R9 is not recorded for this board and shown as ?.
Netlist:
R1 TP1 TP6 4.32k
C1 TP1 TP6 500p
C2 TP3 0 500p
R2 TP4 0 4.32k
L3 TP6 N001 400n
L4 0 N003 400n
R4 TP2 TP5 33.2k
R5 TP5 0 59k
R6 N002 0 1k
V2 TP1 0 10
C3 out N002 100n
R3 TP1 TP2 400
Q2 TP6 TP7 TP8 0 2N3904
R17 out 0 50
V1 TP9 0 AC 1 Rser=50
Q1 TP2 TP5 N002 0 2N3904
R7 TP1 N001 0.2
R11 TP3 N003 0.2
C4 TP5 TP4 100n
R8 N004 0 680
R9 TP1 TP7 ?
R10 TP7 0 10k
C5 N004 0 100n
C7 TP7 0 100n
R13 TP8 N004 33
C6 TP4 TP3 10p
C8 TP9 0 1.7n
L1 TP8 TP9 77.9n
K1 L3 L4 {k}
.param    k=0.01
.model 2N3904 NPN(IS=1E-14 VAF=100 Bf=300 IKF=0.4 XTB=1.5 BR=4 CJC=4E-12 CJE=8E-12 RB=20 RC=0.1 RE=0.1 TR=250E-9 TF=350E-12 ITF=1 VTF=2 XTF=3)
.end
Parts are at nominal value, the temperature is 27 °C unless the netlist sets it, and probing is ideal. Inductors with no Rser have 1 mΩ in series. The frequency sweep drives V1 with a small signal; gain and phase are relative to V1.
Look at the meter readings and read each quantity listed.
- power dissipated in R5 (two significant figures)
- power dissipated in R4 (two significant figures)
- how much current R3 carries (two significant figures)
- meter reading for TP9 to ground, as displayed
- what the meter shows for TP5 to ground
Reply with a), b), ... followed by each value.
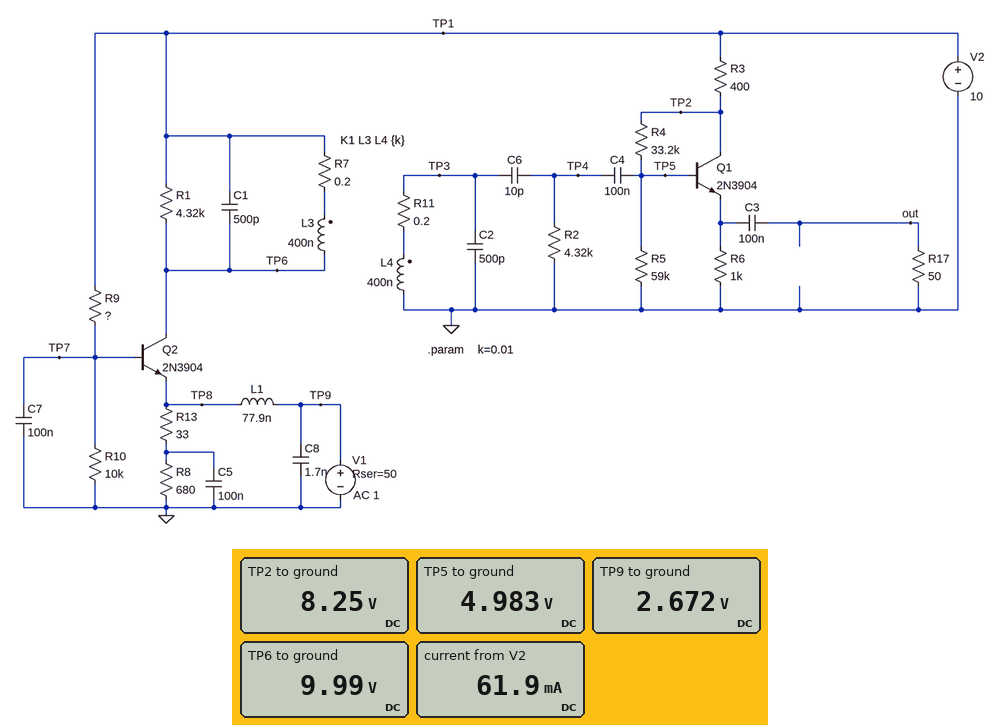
a) 420 µW
b) 320 µW
c) 4.4 mA
d) 2.672 V
e) 4.983 V
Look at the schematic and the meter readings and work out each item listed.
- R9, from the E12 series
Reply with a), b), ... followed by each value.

a) 12 kΩ
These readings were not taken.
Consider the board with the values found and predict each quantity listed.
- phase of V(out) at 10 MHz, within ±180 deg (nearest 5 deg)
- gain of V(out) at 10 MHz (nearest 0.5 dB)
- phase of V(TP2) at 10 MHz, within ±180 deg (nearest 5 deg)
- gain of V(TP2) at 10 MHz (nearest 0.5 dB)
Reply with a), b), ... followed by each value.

a) -100 deg
b) -24.5 dB
c) 75 deg
d) -6.0 dB
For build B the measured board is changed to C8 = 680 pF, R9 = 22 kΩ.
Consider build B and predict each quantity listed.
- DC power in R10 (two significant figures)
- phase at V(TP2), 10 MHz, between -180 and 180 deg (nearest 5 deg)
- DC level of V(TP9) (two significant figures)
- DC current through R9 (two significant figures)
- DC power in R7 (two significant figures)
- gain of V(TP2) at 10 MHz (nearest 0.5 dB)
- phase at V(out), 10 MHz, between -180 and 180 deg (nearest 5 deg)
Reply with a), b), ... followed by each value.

a) 550 µW
b) 85 deg
c) 1.6 V
d) 350 µA
e) 230 µW
f) -11.0 dB
g) -90 deg
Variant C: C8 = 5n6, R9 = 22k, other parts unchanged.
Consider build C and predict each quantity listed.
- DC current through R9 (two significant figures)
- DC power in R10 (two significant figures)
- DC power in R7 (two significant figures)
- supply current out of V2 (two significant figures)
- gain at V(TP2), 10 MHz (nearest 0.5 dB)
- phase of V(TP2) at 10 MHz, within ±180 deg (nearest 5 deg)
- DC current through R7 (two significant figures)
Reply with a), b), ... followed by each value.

a) 350 µA
b) 550 µW
c) 230 µW
d) 39 mA
e) -12.5 dB
f) -65 deg
g) 34 mA
